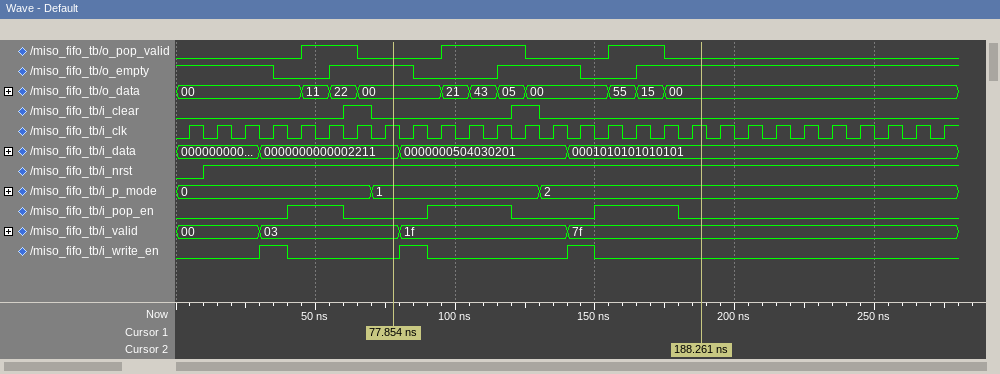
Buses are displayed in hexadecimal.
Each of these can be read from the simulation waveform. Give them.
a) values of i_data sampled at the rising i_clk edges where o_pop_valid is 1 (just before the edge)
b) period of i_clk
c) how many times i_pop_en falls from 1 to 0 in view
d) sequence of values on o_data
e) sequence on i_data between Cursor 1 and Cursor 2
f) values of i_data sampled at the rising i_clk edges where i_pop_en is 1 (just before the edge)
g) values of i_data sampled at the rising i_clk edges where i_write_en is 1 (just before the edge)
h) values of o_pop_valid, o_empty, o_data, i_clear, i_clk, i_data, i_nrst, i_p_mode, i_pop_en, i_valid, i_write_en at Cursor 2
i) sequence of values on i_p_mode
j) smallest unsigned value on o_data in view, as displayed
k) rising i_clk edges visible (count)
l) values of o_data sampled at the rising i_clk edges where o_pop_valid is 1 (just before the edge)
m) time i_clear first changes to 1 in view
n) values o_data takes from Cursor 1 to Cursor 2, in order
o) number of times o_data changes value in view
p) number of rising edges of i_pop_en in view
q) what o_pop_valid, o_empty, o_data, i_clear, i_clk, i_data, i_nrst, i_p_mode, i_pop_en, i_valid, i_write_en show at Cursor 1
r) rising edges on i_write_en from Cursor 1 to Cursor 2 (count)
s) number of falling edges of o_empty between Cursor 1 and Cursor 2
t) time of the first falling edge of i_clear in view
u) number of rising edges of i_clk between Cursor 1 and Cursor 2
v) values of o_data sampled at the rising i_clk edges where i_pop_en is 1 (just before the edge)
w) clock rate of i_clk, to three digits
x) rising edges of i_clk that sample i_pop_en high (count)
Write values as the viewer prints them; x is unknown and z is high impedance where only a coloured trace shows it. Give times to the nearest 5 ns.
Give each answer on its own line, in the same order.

0000000000002211, 0000000000002211, 0000000504030201, 0000000504030201, 0000000504030201, 0001010101010101, 0001010101010101
10 ns
3
00, 11, 22, 00, 21, 43, 05, 00, 55, 15, 00
0000000000002211, 0000000504030201, 0001010101010101
0000000000002211, 0000000000002211, 0000000504030201, 0000000504030201, 0000000504030201, 0001010101010101, 0001010101010101, 0001010101010101
0000000000002211, 0000000504030201, 0001010101010101
o_pop_valid=0, o_empty=1, o_data=00, i_clear=0, i_clk=1, i_data=0001010101010101, i_nrst=1, i_p_mode=2, i_pop_en=0, i_valid=7f, i_write_en=0
0, 1, 2
00
28
11, 22, 21, 43, 05, 55, 15
60 ns
00, 21, 43, 05, 00, 55, 15, 00
10
3
o_pop_valid=0, o_empty=1, o_data=00, i_clear=0, i_clk=1, i_data=0000000000002211, i_nrst=1, i_p_mode=1, i_pop_en=0, i_valid=03, i_write_en=0
2
2
70 ns
11
00, 11, 00, 21, 43, 00, 55, 15
100 MHz
8
